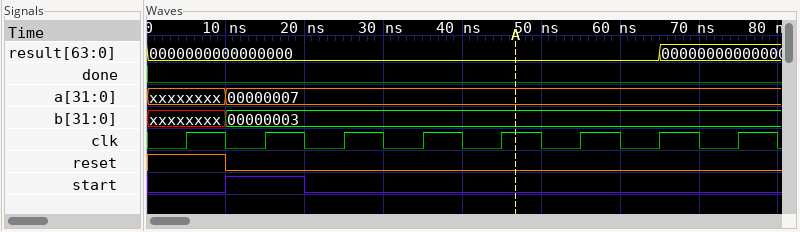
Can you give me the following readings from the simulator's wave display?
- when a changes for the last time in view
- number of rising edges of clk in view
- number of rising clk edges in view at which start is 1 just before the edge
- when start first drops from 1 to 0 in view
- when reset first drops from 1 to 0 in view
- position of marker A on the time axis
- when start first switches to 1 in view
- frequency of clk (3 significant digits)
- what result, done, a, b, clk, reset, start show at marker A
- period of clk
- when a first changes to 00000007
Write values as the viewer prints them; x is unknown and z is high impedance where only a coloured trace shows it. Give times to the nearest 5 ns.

10 ns
8
1
20 ns
10 ns
45 ns
10 ns
100 MHz
result=0000000000000000, done=0, a=00000007, b=00000003, clk=1, reset=0, start=0
10 ns
10 ns
